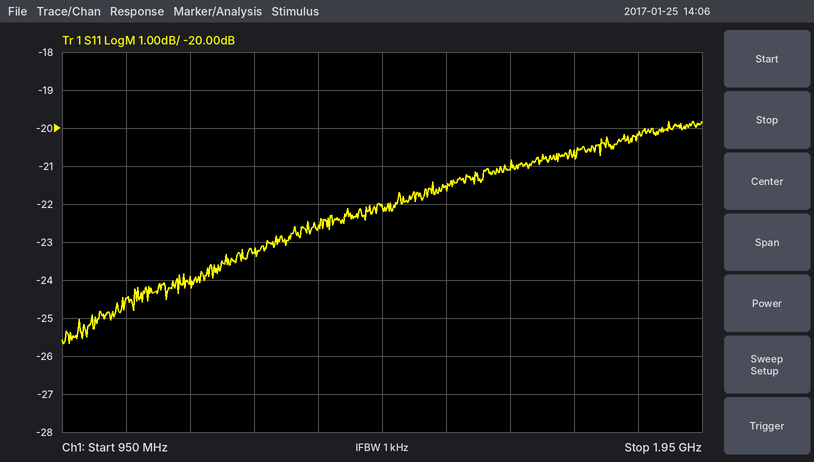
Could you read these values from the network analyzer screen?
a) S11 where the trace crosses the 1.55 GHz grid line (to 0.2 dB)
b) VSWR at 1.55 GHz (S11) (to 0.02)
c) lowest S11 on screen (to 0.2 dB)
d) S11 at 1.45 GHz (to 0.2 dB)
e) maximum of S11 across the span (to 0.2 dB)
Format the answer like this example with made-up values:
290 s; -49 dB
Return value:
-21.6 dB; 1.18; -25.6 dB; -22.0 dB; -19.8 dB
